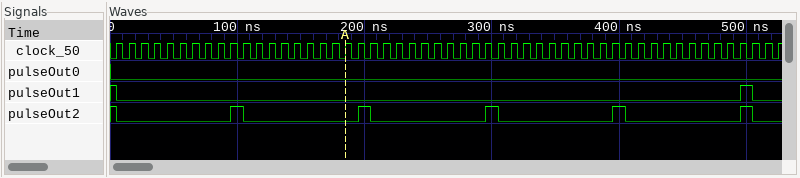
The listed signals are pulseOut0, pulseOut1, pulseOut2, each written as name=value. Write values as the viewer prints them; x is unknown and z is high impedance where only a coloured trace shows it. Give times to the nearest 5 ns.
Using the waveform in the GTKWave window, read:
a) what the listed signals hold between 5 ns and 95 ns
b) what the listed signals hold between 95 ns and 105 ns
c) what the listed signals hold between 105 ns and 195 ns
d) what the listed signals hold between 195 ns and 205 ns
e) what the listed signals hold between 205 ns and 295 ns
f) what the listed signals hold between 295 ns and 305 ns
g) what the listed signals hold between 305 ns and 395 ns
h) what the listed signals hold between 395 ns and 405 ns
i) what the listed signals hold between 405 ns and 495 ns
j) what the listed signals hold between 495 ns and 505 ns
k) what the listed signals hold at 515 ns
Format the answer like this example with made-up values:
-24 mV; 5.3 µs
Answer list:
pulseOut0=0, pulseOut1=0, pulseOut2=0; pulseOut0=0, pulseOut1=0, pulseOut2=1; pulseOut0=0, pulseOut1=0, pulseOut2=0; pulseOut0=0, pulseOut1=0, pulseOut2=1; pulseOut0=0, pulseOut1=0, pulseOut2=0; pulseOut0=0, pulseOut1=0, pulseOut2=1; pulseOut0=0, pulseOut1=0, pulseOut2=0; pulseOut0=0, pulseOut1=0, pulseOut2=1; pulseOut0=0, pulseOut1=0, pulseOut2=0; pulseOut0=0, pulseOut1=1, pulseOut2=1; pulseOut0=0, pulseOut1=0, pulseOut2=0
